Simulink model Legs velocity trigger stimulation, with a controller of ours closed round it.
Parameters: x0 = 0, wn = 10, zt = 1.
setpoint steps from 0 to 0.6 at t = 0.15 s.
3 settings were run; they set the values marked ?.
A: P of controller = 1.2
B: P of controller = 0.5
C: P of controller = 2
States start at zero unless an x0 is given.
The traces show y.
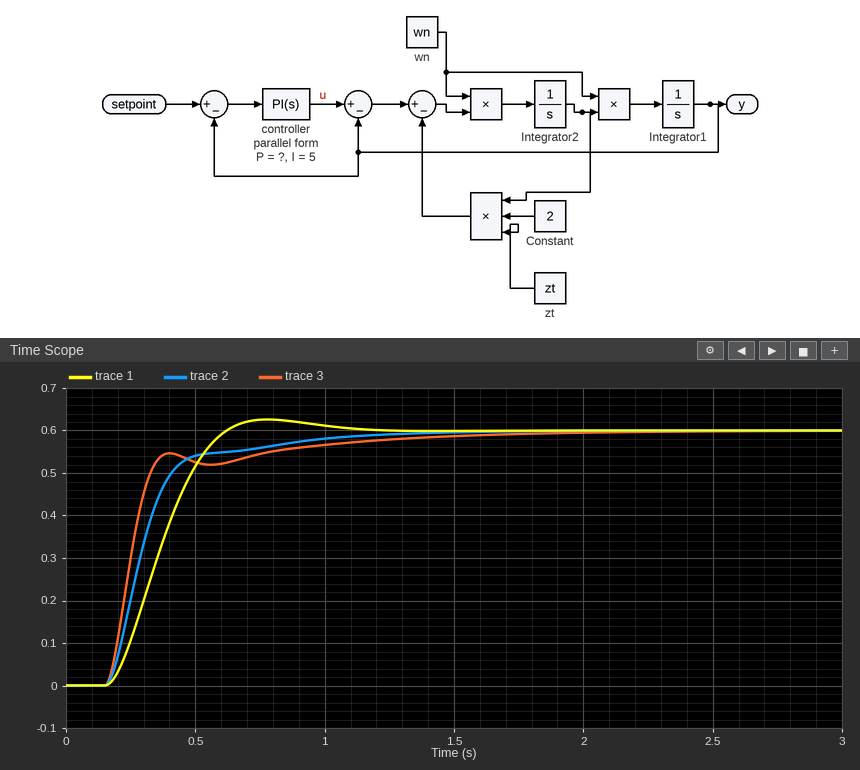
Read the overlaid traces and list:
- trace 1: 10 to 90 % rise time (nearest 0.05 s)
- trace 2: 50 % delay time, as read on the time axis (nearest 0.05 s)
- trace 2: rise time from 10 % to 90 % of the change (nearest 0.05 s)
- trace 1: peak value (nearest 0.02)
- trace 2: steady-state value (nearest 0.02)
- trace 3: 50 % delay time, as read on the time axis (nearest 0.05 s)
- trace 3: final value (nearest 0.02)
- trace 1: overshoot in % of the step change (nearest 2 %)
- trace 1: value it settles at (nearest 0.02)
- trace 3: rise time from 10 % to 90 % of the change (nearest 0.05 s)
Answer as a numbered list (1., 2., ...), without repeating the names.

1. 0.30 s
2. 0.30 s
3. 0.30 s
4. 0.62
5. 0.60
6. 0.25 s
7. 0.60
8. 4 %
9. 0.60
10. 0.20 s
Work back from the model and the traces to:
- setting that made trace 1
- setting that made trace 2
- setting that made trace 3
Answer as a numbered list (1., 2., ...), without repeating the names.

1. B
2. A
3. C
